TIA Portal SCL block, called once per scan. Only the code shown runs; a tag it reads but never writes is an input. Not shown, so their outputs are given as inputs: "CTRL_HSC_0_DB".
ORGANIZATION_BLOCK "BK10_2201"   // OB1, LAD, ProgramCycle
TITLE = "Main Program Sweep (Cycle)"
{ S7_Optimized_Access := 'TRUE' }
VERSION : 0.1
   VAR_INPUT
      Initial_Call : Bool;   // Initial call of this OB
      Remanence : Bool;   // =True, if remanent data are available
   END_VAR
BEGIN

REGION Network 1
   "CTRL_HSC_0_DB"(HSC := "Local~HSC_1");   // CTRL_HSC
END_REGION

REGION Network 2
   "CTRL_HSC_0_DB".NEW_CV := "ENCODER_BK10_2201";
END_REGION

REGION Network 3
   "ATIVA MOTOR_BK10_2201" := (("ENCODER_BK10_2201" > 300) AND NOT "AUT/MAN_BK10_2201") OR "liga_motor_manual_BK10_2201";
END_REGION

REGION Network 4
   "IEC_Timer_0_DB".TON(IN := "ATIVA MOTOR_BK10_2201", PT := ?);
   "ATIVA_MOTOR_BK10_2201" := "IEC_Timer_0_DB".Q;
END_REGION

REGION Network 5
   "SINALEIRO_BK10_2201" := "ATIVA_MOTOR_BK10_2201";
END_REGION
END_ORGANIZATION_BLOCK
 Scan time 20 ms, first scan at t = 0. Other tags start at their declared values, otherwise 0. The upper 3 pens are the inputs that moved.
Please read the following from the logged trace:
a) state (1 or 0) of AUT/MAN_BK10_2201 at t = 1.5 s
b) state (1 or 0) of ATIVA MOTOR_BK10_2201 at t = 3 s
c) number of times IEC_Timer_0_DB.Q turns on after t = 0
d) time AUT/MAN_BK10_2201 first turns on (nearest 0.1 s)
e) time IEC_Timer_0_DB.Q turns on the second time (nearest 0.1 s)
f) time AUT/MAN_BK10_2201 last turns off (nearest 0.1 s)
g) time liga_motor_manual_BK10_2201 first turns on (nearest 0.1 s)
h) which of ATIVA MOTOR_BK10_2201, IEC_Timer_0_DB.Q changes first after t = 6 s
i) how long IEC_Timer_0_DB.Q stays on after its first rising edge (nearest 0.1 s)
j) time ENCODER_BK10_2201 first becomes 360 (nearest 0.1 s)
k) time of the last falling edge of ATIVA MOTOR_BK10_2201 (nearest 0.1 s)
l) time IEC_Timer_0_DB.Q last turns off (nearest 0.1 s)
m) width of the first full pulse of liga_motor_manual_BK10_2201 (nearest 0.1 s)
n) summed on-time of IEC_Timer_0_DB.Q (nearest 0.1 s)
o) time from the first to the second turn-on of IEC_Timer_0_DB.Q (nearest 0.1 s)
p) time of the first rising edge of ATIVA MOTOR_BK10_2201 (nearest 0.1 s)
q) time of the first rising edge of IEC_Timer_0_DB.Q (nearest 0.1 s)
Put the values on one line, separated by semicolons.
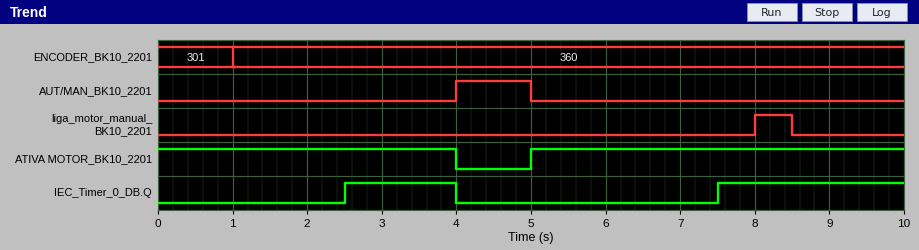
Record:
0; 1; 2; 4.0 s; 7.5 s; 5.0 s; 8.0 s; IEC_Timer_0_DB.Q; 1.5 s; 1.0 s; 4.0 s; 4.0 s; 0.5 s; 4.0 s; 5.0 s; 5.0 s; 2.5 s
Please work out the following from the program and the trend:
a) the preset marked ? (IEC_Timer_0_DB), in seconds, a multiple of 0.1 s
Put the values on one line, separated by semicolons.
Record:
2.5 s
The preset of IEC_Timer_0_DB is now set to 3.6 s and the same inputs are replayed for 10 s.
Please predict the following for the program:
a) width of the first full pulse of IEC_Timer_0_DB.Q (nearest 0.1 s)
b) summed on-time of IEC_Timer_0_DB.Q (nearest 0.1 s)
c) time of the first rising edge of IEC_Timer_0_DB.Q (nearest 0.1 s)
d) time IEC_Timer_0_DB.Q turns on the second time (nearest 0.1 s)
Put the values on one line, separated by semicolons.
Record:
0.4 s; 1.8 s; 3.6 s; 8.6 s
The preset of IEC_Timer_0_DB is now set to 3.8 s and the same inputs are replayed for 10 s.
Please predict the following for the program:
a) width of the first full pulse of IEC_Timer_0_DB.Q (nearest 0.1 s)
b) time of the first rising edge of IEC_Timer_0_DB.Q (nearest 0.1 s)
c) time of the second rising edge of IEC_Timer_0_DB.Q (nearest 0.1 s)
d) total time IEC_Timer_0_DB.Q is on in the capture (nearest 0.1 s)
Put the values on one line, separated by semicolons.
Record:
0.2 s; 3.8 s; 8.8 s; 1.4 s
